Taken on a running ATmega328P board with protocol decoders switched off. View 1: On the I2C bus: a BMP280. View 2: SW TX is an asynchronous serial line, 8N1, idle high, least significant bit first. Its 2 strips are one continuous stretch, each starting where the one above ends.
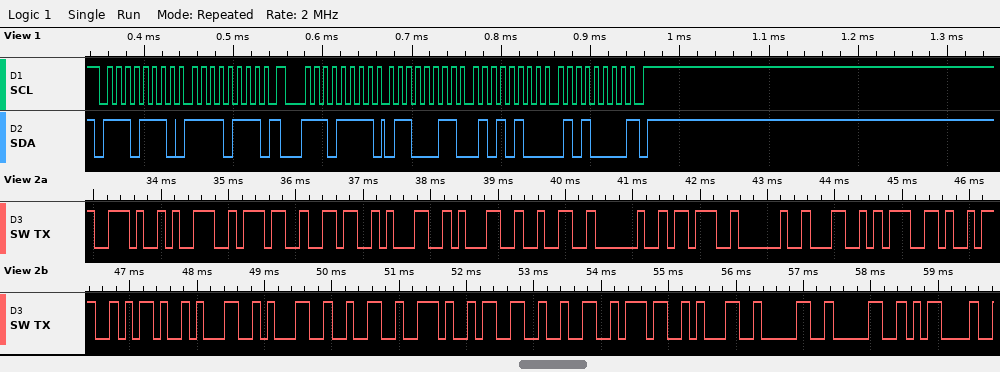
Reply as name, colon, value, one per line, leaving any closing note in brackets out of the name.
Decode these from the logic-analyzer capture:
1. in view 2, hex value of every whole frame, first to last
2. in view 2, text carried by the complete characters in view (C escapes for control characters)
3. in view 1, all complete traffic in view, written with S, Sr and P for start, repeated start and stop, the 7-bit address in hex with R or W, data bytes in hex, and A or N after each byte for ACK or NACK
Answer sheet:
in view 2, hex value of every whole frame, first to last: 2E 39 37 36 31 31 32 20 3B 20 4C 67 3A 2D 31 31 32 2E 33 32 37 31 30 30 0D
in view 2, text carried by the complete characters in view: ".976112 ; Lg:-112.327100\r"
in view 1, all complete traffic in view, written with S, Sr and P for start, repeated start and stop, the 7-bit address in hex with R or W, data bytes in hex, and A or N after each byte for ACK or NACK: S 77W A F7 A Sr 77R A 63 A 54 A 50 N P
